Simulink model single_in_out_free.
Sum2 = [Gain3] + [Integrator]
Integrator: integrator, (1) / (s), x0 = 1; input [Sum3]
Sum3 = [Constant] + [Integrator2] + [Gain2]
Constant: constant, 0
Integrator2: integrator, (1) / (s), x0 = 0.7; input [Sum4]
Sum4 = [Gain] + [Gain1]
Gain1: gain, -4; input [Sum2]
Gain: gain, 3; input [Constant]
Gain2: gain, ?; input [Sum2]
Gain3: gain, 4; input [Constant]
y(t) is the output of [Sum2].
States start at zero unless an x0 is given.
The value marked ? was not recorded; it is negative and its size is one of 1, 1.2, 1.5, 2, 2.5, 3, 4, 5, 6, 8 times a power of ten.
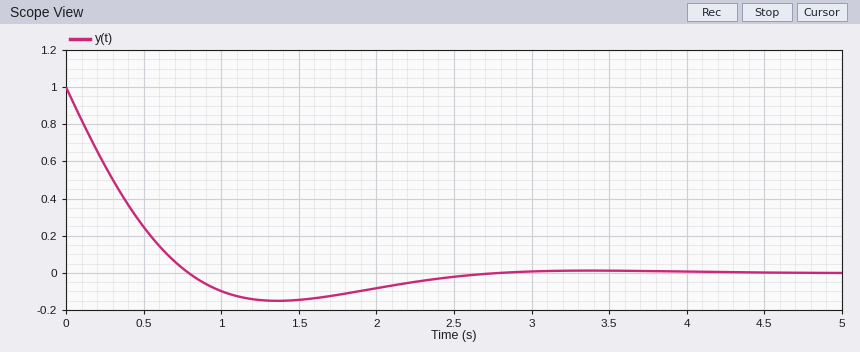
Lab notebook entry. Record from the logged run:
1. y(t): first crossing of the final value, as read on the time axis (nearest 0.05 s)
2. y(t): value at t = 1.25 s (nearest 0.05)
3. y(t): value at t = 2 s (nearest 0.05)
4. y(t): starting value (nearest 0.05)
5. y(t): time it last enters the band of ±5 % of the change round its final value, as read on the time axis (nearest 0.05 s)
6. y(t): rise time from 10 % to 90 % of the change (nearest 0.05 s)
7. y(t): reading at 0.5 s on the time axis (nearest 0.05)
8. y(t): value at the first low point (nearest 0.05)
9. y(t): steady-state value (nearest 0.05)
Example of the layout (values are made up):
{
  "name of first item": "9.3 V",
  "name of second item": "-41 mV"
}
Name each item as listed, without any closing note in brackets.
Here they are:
{
  "y(t): first crossing of the final value, as read on the time axis": "0.80 s",
  "y(t): value at t = 1.25 s": "-0.15",
  "y(t): value at t = 2 s": "-0.10",
  "y(t): starting value": "1.00",
  "y(t): time it last enters the band of ±5 % of the change round its final value, as read on the time axis": "2.25 s",
  "y(t): rise time from 10 % to 90 % of the change": "0.60 s",
  "y(t): reading at 0.5 s on the time axis": "0.25",
  "y(t): value at the first low point": "-0.15",
  "y(t): steady-state value": "0.00"
}
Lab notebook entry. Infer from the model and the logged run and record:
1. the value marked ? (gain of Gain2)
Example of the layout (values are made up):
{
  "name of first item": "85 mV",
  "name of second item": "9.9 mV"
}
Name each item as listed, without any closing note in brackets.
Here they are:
{
  "the value marked ?": "-2.5"
}
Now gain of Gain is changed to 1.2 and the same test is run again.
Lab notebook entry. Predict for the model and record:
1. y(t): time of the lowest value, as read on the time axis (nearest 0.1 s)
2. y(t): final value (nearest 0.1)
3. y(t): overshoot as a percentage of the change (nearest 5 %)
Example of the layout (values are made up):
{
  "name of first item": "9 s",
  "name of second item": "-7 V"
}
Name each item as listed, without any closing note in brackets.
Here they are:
{
  "y(t): time of the lowest value, as read on the time axis": "1.4 s",
  "y(t): final value": "0.0",
  "y(t): overshoot as a percentage of the change": "15 %"
}
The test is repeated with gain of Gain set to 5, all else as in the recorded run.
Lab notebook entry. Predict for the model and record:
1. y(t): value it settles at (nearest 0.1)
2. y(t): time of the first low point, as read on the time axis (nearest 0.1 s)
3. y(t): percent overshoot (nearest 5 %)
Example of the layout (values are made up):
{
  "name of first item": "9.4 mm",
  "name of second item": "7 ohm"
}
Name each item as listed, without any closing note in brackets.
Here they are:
{
  "y(t): value it settles at": "0.0",
  "y(t): time of the first low point, as read on the time axis": "1.4 s",
  "y(t): percent overshoot": "15 %"
}
